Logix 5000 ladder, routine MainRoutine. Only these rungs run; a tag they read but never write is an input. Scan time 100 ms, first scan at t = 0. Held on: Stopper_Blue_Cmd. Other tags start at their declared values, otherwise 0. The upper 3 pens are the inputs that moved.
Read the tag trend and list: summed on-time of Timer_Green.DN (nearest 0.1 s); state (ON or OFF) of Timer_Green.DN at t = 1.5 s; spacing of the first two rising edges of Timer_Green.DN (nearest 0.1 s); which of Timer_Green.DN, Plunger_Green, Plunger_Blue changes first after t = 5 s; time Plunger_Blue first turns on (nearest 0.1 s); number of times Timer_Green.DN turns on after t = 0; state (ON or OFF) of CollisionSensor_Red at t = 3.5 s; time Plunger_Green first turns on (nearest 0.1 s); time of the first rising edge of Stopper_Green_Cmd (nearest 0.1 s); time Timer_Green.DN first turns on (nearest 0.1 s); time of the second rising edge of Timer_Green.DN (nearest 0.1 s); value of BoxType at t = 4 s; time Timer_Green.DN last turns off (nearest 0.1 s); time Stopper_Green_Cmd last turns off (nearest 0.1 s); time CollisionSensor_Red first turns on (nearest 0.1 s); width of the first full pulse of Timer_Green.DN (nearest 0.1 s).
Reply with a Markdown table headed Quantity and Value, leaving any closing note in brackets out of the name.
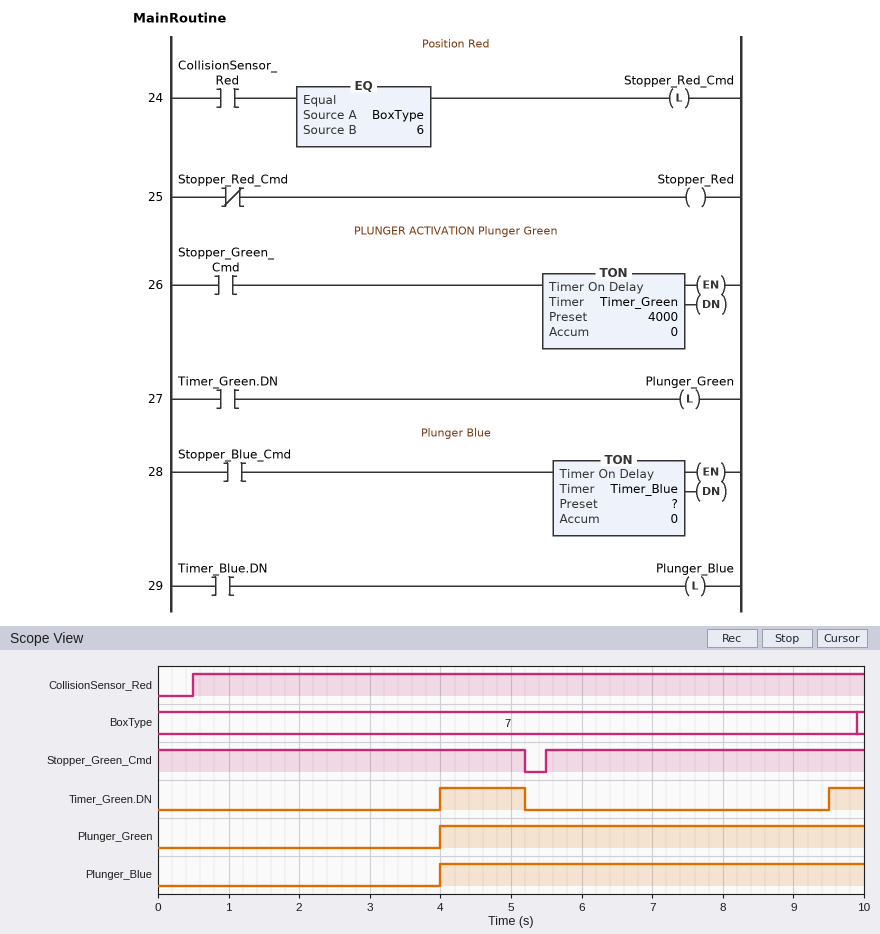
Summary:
| Quantity | Value |
|---|---|
| summed on-time of Timer_Green.DN | 1.7 s |
| state (ON or OFF) of Timer_Green.DN at t = 1.5 s | OFF |
| spacing of the first two rising edges of Timer_Green.DN | 5.5 s |
| which of Timer_Green.DN, Plunger_Green, Plunger_Blue changes first after t = 5 s | Timer_Green.DN |
| time Plunger_Blue first turns on | 4.0 s |
| number of times Timer_Green.DN turns on after t = 0 | 2 |
| state (ON or OFF) of CollisionSensor_Red at t = 3.5 s | ON |
| time Plunger_Green first turns on | 4.0 s |
| time of the first rising edge of Stopper_Green_Cmd | 5.5 s |
| time Timer_Green.DN first turns on | 4.0 s |
| time of the second rising edge of Timer_Green.DN | 9.5 s |
| value of BoxType at t = 4 s | 7 |
| time Timer_Green.DN last turns off | 5.2 s |
| time Stopper_Green_Cmd last turns off | 5.2 s |
| time CollisionSensor_Red first turns on | 0.5 s |
| width of the first full pulse of Timer_Green.DN | 1.2 s |
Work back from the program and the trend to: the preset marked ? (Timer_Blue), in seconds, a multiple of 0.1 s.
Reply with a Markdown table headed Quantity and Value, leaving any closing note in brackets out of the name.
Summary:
| Quantity | Value |
|---|---|
| the preset marked ? (Timer_Blue), in seconds, a multiple of 0.1 s | 4.0 s |
